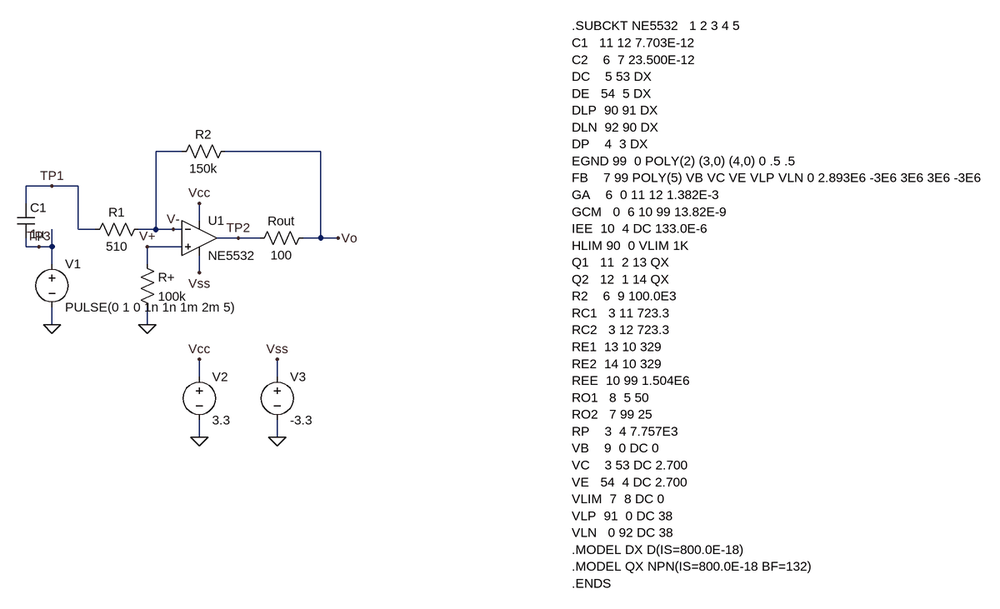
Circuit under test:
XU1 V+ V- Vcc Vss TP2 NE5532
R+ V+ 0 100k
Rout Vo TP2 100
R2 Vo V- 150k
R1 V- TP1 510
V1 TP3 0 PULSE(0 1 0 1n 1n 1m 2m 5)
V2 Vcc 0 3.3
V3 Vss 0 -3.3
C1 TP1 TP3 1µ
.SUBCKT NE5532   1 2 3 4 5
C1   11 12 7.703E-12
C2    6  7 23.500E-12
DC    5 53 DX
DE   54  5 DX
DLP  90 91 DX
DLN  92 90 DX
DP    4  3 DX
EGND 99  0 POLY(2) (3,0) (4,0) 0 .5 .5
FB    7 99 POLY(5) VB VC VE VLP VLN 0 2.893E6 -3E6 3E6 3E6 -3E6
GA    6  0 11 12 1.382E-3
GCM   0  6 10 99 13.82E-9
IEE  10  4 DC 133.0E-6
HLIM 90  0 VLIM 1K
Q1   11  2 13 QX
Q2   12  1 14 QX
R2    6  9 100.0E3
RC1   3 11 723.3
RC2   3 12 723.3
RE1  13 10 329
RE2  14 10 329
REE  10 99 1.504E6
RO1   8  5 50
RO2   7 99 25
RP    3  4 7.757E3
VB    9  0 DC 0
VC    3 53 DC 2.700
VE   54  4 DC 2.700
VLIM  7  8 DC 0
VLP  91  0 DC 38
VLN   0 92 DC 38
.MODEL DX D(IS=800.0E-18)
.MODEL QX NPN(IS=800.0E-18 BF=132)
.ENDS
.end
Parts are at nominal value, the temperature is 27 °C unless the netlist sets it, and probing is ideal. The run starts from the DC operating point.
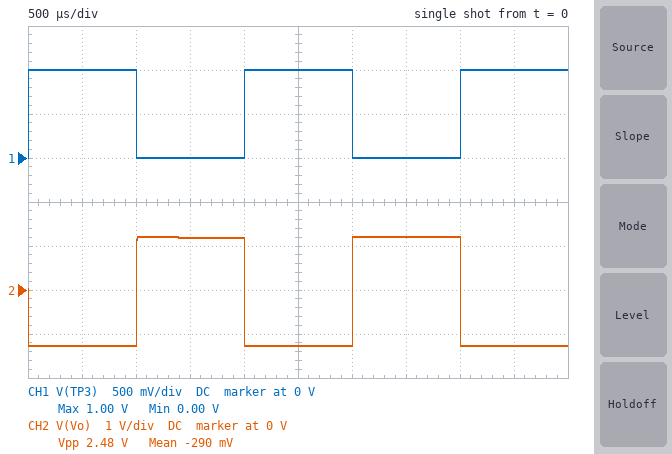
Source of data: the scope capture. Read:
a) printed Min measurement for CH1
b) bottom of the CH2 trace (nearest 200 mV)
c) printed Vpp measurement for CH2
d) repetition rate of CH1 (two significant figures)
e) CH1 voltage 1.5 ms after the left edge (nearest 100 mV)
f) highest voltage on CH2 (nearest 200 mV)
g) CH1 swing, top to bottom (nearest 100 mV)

0.00 V
-1.2 V
2.48 V
500 Hz
0 V
1.2 V
1.0 V
